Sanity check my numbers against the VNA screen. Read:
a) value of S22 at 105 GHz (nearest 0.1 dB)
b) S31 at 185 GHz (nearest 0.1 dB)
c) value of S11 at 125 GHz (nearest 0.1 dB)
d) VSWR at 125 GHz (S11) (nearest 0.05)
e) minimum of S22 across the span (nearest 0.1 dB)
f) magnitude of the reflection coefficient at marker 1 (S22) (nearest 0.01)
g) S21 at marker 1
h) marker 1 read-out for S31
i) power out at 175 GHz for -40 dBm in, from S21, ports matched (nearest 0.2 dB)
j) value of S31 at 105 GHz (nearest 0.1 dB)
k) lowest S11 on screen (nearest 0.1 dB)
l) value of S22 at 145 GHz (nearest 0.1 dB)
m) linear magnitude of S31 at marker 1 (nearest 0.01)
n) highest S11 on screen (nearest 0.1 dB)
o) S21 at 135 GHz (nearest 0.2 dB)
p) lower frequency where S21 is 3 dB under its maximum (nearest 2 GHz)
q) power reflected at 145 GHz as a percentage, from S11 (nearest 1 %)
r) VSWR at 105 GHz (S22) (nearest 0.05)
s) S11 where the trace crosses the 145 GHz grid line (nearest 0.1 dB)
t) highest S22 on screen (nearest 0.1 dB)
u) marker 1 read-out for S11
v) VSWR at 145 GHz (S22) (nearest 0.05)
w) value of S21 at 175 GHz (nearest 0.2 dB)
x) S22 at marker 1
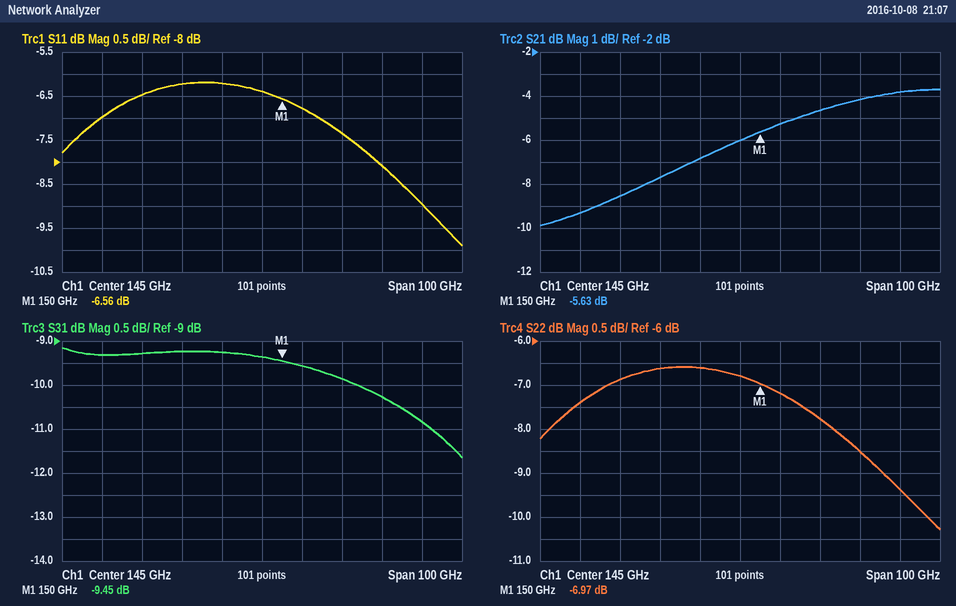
-7.4 dB
-10.8 dB
-6.2 dB
2.90
-10.3 dB
0.45
-5.63 dB
-9.45 dB
-44.2 dBm
-9.3 dB
-9.9 dB
-6.8 dB
0.34
-6.2 dB
-6.8 dB
136 GHz
23 %
2.50
-6.4 dB
-6.6 dB
-6.56 dB
2.70
-4.2 dB
-6.97 dB
